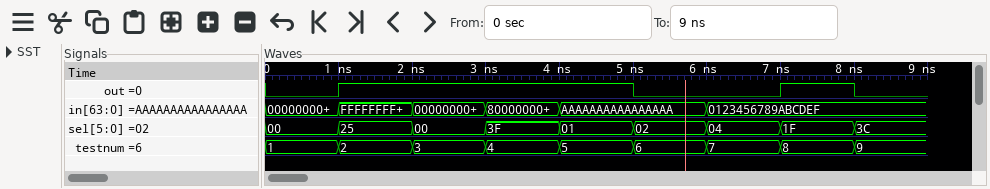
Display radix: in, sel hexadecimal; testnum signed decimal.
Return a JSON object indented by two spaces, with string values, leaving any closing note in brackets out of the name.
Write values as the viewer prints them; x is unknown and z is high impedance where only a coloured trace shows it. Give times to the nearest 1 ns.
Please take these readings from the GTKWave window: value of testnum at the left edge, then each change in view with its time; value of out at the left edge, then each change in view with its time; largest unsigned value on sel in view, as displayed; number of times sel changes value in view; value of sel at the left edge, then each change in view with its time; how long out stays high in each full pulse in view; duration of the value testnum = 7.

{
  "value of testnum at the left edge, then each change in view with its time": "1, 2 at 1 ns, 3 at 2 ns, 4 at 3 ns, 5 at 4 ns, 6 at 5 ns, 7 at 6 ns, 8 at 7 ns, 9 at 8 ns",
  "value of out at the left edge, then each change in view with its time": "0, 1 at 1 ns, 0 at 5 ns, 1 at 7 ns, 0 at 8 ns",
  "largest unsigned value on sel in view, as displayed": "3F",
  "number of times sel changes value in view": "8",
  "value of sel at the left edge, then each change in view with its time": "00, 25 at 1 ns, 00 at 2 ns, 3F at 3 ns, 01 at 4 ns, 02 at 5 ns, 04 at 6 ns, 1F at 7 ns, 3C at 8 ns",
  "how long out stays high in each full pulse in view": "4 ns, 1 ns",
  "duration of the value testnum = 7": "1 ns"
}
